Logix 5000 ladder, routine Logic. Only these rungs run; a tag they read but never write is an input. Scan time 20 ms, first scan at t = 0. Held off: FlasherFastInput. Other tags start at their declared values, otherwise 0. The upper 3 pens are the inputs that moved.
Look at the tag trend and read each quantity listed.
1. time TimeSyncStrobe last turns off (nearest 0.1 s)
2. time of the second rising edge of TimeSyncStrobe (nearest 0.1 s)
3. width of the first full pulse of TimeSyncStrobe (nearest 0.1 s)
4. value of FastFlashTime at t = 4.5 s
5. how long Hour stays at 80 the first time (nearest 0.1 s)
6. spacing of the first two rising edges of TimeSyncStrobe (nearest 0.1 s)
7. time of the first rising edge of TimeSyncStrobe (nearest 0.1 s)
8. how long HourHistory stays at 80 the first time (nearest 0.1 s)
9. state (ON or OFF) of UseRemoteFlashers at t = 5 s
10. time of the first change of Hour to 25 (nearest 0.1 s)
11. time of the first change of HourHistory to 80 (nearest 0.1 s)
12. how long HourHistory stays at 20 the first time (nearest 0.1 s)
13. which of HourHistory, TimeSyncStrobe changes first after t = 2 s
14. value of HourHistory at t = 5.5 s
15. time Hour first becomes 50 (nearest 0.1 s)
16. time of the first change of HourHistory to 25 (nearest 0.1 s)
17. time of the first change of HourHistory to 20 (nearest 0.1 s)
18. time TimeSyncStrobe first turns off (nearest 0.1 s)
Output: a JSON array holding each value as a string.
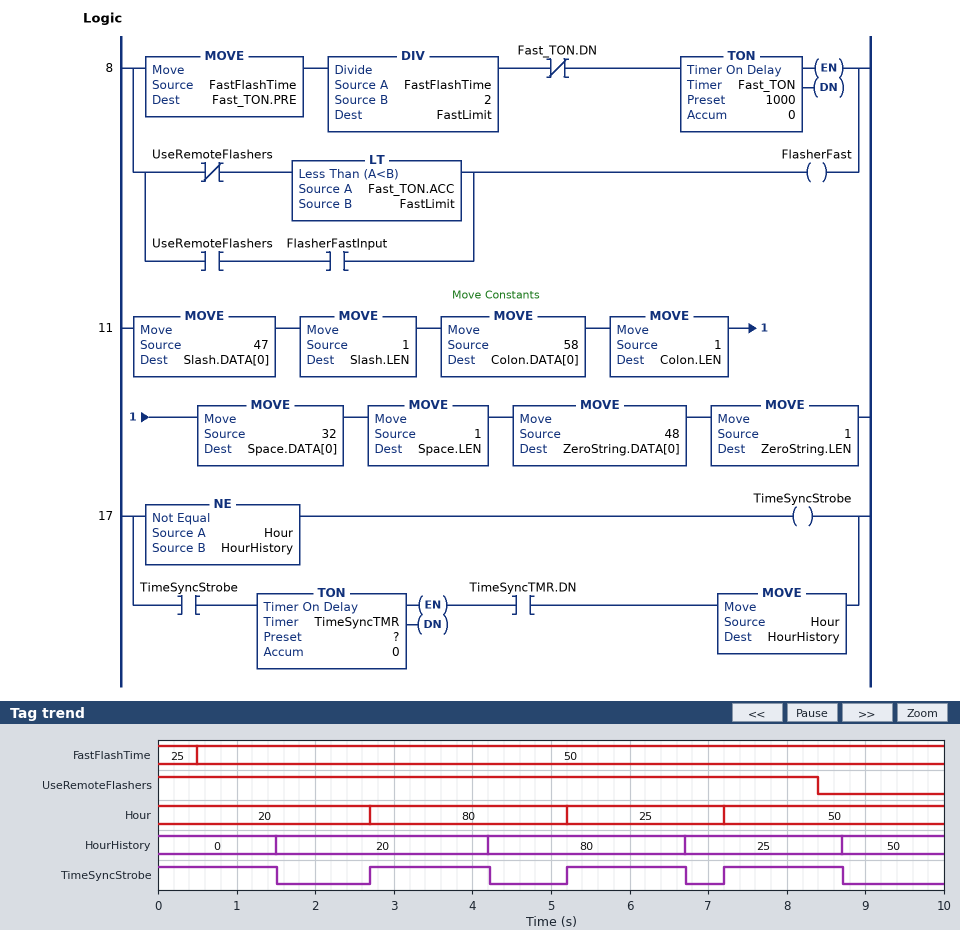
["8.7 s", "5.2 s", "1.5 s", "50", "2.5 s", "2.5 s", "2.7 s", "2.5 s", "ON", "5.2 s", "4.2 s", "2.7 s", "TimeSyncStrobe", "80", "7.2 s", "6.7 s", "1.5 s", "1.5 s"]
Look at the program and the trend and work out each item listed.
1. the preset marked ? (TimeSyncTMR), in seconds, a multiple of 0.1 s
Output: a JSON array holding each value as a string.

["1.5 s"]
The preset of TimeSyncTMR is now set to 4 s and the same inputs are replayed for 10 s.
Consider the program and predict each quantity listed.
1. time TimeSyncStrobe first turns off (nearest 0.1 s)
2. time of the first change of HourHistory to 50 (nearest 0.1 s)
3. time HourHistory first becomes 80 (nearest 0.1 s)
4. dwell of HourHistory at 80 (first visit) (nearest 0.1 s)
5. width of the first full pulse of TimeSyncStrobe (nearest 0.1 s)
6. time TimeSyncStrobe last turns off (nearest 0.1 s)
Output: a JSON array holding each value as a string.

["4.0 s", "9.2 s", "4.0 s", "5.2 s", "4.0 s", "9.2 s"]
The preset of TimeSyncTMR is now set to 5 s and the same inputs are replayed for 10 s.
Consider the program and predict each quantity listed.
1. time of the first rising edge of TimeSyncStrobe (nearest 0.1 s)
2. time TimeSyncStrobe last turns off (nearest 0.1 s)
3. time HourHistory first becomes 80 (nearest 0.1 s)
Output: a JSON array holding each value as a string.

["5.2 s", "5.0 s", "5.0 s"]
